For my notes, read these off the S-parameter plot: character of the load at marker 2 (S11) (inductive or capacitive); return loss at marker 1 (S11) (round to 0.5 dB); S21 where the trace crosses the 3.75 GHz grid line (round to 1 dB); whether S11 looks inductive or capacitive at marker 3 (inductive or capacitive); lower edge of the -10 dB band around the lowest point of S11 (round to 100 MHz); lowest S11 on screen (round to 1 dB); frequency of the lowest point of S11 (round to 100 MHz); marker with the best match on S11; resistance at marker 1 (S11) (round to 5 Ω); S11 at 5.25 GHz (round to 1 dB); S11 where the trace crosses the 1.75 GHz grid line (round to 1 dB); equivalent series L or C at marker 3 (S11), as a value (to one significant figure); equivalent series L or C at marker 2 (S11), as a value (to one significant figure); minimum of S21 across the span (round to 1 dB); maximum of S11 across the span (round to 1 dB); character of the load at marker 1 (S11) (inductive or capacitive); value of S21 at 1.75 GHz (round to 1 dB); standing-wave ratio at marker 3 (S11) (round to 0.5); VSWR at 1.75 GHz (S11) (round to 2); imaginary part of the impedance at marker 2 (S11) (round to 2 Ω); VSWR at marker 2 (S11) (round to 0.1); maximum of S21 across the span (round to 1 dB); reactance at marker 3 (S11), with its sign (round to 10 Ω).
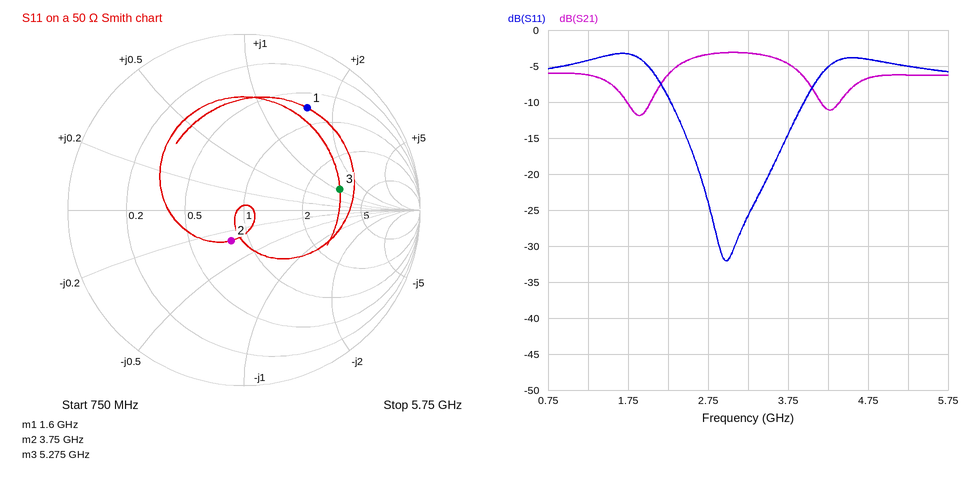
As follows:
capacitive
3.5 dB
-5 dB
inductive
2.3 GHz
-32 dB
3.0 GHz
marker 2
35 Ω
-5 dB
-3 dB
2 nH
3 pF
-12 dB
-3 dB
inductive
-10 dB
3.5
6
-14 Ω
1.5
-3 dB
+50 Ω
